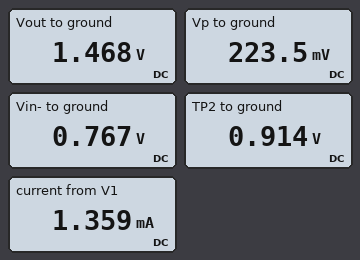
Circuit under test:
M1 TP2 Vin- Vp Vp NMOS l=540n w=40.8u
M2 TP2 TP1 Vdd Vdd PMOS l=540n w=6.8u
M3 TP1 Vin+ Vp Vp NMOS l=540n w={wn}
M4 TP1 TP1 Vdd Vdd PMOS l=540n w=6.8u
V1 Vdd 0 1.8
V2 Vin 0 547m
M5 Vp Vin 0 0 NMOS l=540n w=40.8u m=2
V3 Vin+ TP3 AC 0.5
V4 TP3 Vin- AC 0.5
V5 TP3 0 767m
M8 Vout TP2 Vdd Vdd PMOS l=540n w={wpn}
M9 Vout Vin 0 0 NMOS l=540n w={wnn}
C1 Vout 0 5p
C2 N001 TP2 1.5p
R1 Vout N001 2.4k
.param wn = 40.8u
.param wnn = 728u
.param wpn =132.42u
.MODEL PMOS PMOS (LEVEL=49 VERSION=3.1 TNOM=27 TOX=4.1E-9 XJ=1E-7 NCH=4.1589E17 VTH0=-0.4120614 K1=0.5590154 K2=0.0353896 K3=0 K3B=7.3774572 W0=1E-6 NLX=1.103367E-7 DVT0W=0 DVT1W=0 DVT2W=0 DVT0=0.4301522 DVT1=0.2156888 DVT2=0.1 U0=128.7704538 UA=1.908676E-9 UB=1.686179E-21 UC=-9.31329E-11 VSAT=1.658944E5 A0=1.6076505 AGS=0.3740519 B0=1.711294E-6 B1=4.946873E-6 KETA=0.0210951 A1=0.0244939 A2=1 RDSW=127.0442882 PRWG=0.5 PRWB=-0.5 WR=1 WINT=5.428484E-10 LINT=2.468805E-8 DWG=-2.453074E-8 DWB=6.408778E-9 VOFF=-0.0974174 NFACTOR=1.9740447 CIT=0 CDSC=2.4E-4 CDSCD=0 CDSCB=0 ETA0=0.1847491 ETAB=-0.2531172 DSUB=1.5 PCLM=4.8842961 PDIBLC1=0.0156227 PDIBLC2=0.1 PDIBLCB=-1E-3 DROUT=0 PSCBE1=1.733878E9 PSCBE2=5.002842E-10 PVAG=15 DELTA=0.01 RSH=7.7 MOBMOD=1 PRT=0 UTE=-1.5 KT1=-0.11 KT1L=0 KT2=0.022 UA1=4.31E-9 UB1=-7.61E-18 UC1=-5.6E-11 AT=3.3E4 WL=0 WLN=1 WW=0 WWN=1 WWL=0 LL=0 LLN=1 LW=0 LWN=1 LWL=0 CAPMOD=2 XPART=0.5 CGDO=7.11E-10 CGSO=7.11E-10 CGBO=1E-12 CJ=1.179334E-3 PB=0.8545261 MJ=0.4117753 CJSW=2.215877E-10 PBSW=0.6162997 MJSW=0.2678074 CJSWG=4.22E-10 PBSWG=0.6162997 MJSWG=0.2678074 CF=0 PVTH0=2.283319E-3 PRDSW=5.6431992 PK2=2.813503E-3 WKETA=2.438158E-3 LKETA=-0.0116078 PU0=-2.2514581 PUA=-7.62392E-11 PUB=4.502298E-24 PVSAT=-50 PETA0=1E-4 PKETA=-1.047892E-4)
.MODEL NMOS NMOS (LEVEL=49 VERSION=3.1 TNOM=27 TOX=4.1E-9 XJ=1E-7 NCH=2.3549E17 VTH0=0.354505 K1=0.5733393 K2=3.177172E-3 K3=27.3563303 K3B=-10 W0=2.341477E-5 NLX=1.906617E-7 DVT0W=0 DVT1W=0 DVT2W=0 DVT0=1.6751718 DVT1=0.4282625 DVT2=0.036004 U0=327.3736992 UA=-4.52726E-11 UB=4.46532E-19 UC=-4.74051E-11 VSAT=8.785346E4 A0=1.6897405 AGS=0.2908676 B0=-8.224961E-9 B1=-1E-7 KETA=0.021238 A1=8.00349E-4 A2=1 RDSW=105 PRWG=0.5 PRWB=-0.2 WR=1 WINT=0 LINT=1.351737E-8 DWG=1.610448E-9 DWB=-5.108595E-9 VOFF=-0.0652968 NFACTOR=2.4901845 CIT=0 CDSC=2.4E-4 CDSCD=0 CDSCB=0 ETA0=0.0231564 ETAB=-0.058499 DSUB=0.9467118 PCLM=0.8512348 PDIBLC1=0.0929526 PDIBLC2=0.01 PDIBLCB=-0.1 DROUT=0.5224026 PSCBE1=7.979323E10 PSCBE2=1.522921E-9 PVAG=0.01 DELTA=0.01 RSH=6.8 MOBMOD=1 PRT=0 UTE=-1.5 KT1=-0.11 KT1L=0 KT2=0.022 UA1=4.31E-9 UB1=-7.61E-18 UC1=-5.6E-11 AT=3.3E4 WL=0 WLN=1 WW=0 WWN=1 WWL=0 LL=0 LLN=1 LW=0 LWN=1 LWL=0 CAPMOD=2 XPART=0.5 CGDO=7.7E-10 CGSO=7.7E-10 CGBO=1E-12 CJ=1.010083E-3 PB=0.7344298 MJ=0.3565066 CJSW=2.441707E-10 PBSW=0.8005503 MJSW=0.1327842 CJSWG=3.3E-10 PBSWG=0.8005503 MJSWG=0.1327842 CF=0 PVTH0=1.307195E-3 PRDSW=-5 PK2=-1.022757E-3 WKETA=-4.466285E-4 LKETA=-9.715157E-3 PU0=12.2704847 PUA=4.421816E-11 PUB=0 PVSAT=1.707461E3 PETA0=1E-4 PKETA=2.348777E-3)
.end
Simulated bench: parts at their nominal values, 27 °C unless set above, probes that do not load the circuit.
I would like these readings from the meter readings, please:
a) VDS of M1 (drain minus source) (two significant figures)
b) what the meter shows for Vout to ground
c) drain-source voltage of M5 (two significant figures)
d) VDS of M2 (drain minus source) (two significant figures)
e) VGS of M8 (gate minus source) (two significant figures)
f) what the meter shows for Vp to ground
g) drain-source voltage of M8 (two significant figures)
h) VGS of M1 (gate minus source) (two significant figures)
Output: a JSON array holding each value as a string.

["690 mV", "1.468 V", "220 mV", "-890 mV", "-890 mV", "223.5 mV", "-330 mV", "540 mV"]
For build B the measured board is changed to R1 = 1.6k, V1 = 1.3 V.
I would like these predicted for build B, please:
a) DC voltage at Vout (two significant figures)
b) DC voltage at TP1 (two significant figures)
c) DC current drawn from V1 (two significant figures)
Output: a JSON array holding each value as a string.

["1.0 V", "410 mV", "1.3 mA"]
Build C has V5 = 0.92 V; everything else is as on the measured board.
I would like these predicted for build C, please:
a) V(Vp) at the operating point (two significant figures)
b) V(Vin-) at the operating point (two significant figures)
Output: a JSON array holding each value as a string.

["370 mV", "920 mV"]
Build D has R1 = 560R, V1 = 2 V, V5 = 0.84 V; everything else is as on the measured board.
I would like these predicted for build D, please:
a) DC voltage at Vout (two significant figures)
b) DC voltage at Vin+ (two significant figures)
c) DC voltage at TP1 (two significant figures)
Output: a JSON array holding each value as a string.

["1.7 V", "840 mV", "1.1 V"]
